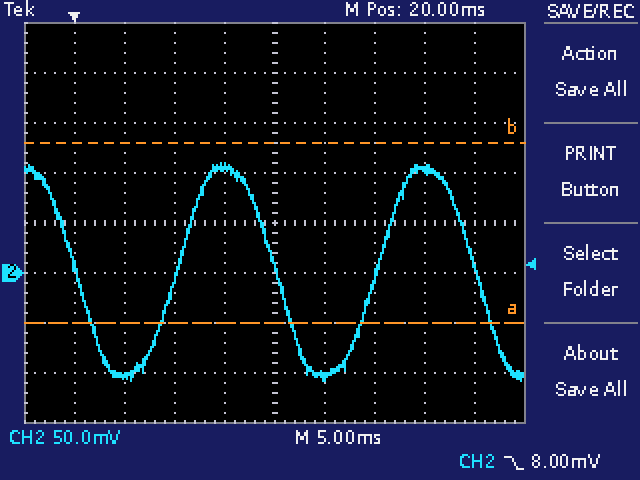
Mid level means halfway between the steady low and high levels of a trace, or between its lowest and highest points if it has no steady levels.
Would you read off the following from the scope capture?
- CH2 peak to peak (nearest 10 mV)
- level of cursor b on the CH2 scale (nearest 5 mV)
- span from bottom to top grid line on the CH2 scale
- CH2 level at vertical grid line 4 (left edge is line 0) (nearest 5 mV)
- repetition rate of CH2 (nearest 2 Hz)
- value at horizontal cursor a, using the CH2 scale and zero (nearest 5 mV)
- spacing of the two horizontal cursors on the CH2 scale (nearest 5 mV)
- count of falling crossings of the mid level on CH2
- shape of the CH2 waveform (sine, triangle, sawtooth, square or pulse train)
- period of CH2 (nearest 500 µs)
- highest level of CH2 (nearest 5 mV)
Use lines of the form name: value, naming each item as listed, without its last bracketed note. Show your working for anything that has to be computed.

CH2 peak to peak: 220 mV
level of cursor b on the CH2 scale: 130 mV
span from bottom to top grid line on the CH2 scale: 400 mV
CH2 level at vertical grid line 4 (left edge is line 0): 105 mV
repetition rate of CH2: 1 / 20.0 ms ≈ 50 Hz
value at horizontal cursor a, using the CH2 scale and zero: -50 mV
spacing of the two horizontal cursors on the CH2 scale: 180 mV
count of falling crossings of the mid level on CH2: 3
shape of the CH2 waveform: sine
period of CH2: 20.0 ms
highest level of CH2: 110 mV
